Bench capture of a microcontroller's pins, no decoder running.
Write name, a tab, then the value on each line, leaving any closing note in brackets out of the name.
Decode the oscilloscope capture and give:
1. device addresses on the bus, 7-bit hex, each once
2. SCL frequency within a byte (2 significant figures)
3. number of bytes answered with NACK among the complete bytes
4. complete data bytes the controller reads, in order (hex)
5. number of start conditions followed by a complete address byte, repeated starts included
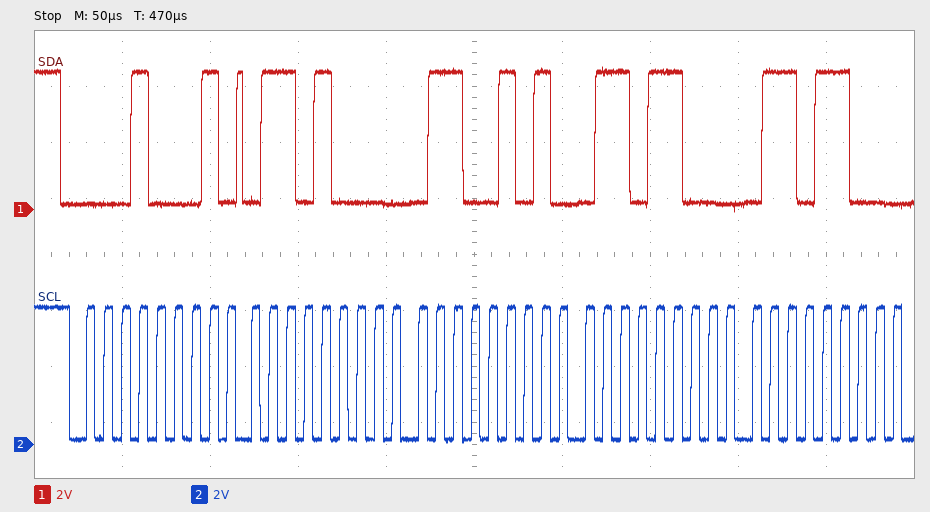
device addresses on the bus, 7-bit hex, each once	0x08
SCL frequency within a byte	100 kHz
number of bytes answered with NACK among the complete bytes	0
complete data bytes the controller reads, in order	68 65 6C 6C
number of start conditions followed by a complete address byte, repeated starts included	1
